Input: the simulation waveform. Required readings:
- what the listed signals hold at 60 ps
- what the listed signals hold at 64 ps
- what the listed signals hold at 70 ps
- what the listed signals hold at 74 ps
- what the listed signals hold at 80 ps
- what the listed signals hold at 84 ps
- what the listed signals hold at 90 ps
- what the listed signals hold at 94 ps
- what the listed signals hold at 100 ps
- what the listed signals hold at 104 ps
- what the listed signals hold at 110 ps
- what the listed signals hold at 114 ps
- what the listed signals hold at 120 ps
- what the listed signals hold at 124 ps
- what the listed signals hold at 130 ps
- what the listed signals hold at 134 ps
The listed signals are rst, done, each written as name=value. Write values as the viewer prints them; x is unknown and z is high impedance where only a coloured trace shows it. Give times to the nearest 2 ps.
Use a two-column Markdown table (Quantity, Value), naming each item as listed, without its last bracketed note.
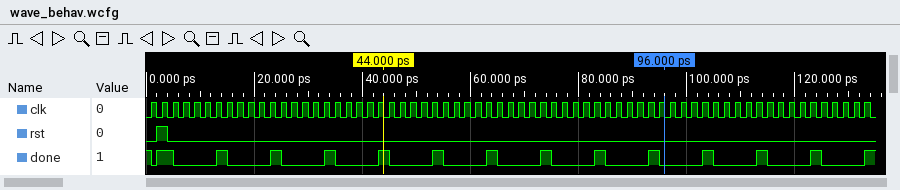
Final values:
| Quantity | Value |
|---|---|
| what the listed signals hold at 60 ps | rst=0, done=0 |
| what the listed signals hold at 64 ps | rst=0, done=1 |
| what the listed signals hold at 70 ps | rst=0, done=0 |
| what the listed signals hold at 74 ps | rst=0, done=1 |
| what the listed signals hold at 80 ps | rst=0, done=0 |
| what the listed signals hold at 84 ps | rst=0, done=1 |
| what the listed signals hold at 90 ps | rst=0, done=0 |
| what the listed signals hold at 94 ps | rst=0, done=1 |
| what the listed signals hold at 100 ps | rst=0, done=0 |
| what the listed signals hold at 104 ps | rst=0, done=1 |
| what the listed signals hold at 110 ps | rst=0, done=0 |
| what the listed signals hold at 114 ps | rst=0, done=1 |
| what the listed signals hold at 120 ps | rst=0, done=0 |
| what the listed signals hold at 124 ps | rst=0, done=1 |
| what the listed signals hold at 130 ps | rst=0, done=0 |
| what the listed signals hold at 134 ps | rst=0, done=1 |
